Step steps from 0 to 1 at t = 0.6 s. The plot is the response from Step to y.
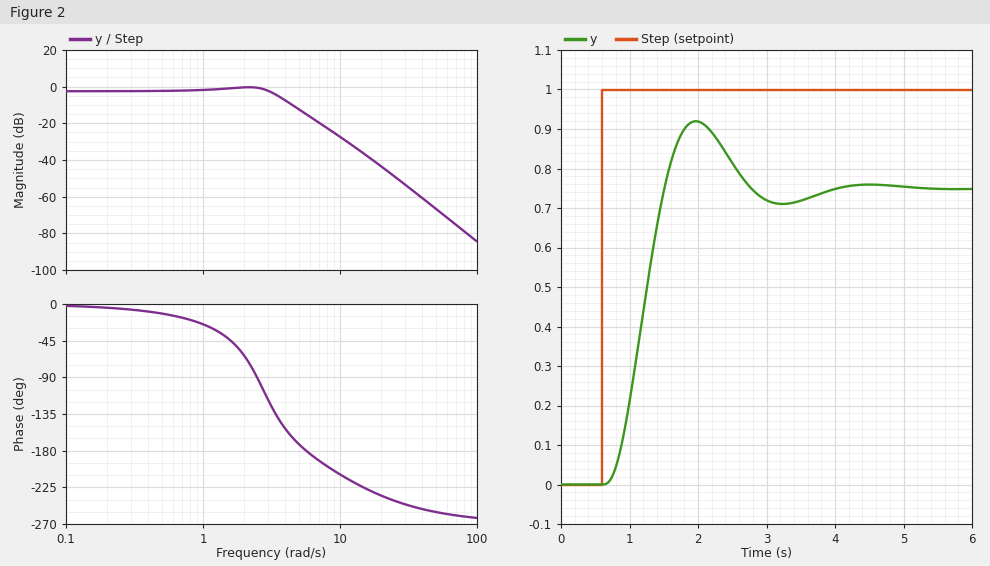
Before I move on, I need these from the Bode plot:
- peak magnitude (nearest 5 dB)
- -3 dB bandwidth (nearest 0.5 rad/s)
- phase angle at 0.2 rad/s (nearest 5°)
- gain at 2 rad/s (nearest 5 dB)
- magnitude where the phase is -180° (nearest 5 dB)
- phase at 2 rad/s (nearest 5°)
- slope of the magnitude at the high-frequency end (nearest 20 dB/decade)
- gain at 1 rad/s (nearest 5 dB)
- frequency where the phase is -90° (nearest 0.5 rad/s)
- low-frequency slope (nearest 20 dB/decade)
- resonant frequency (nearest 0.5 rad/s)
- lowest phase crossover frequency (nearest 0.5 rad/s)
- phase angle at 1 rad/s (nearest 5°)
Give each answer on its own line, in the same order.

0 dB
3.5 rad/s
-5°
0 dB
-15 dB
-65°
-60 dB/decade
0 dB
2.5 rad/s
0 dB/decade
2.0 rad/s
5.5 rad/s
-25°
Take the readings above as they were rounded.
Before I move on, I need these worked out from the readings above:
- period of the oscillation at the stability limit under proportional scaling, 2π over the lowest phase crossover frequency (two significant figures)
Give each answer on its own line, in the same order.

1.1 s
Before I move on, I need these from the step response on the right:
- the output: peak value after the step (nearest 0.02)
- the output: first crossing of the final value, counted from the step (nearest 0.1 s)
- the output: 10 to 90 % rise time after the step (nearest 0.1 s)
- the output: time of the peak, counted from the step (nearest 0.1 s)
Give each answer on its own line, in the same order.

0.92
0.9 s
0.6 s
1.4 s
